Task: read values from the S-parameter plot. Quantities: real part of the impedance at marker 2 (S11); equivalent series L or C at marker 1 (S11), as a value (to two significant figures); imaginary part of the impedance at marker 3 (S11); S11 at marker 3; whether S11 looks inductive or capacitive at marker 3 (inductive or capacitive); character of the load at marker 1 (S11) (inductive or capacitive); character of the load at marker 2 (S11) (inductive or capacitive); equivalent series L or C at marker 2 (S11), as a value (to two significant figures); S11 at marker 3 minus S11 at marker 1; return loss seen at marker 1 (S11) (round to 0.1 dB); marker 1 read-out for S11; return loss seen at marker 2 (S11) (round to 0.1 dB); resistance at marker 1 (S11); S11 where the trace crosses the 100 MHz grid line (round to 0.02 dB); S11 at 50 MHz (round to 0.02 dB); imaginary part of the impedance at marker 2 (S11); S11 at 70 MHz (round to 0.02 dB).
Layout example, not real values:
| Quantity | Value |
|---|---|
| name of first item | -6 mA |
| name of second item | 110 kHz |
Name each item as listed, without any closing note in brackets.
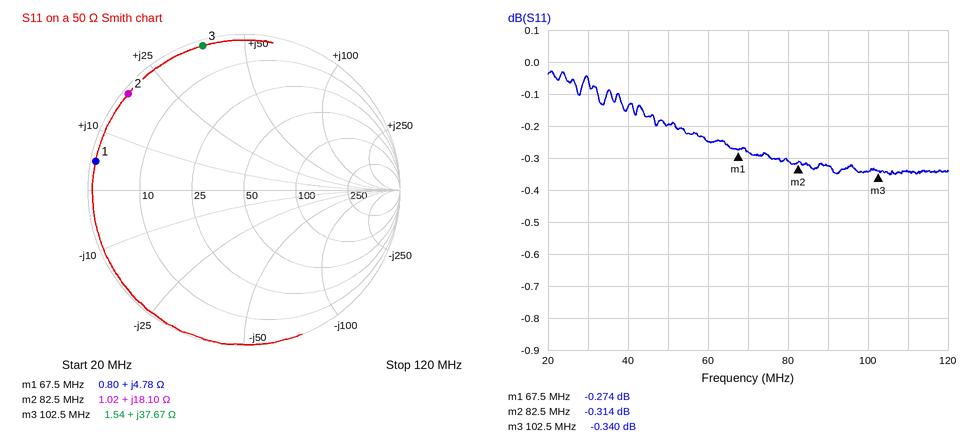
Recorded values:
| Quantity | Value |
|---|---|
| real part of the impedance at marker 2 | 1.02 Ω |
| equivalent series L or C at marker 1 (S11), as a value | 11 nH |
| imaginary part of the impedance at marker 3 | +37.67 Ω |
| S11 at marker 3 | -0.340 dB |
| whether S11 looks inductive or capacitive at marker 3 | inductive |
| character of the load at marker 1 (S11) | inductive |
| character of the load at marker 2 (S11) | inductive |
| equivalent series L or C at marker 2 (S11), as a value | 35 nH |
| S11 at marker 3 minus S11 at marker 1 | -0.066 dB |
| return loss seen at marker 1 (S11) | 0.3 dB |
| marker 1 read-out for S11 | -0.274 dB |
| return loss seen at marker 2 (S11) | 0.3 dB |
| resistance at marker 1 | 0.80 Ω |
| S11 where the trace crosses the 100 MHz grid line | -0.34 dB |
| S11 at 50 MHz | -0.20 dB |
| imaginary part of the impedance at marker 2 | +18.10 Ω |
| S11 at 70 MHz | -0.28 dB |
